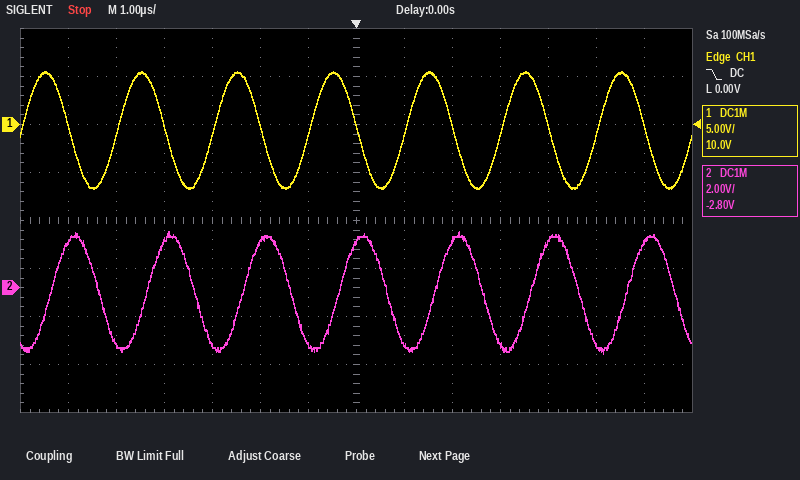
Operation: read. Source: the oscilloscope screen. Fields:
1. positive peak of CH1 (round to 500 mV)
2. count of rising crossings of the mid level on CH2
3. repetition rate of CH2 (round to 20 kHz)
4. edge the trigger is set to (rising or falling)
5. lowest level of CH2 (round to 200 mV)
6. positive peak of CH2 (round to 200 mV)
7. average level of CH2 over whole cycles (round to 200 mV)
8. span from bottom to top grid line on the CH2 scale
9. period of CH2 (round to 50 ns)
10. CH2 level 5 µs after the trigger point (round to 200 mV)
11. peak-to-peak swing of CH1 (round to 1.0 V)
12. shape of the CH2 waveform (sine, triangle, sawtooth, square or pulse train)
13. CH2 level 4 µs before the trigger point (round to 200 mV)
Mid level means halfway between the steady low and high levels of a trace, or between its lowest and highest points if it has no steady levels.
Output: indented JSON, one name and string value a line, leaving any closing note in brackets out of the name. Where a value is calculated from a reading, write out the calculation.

{
  "positive peak of CH1": "5.5 V",
  "count of rising crossings of the mid level on CH2": "7",
  "repetition rate of CH2": "1 / 2.00 µs ≈ 500 kHz",
  "edge the trigger is set to": "falling",
  "lowest level of CH2": "-2.8 V",
  "positive peak of CH2": "2.4 V",
  "average level of CH2 over whole cycles": "(2.4 V + (-2.8 V)) / 2 ≈ -200 mV",
  "span from bottom to top grid line on the CH2 scale": "16 V",
  "period of CH2": "2.00 µs",
  "CH2 level 5 µs after the trigger point": "-2.4 V",
  "peak-to-peak swing of CH1": "12.0 V",
  "shape of the CH2 waveform": "sine",
  "CH2 level 4 µs before the trigger point": "2.0 V"
}
